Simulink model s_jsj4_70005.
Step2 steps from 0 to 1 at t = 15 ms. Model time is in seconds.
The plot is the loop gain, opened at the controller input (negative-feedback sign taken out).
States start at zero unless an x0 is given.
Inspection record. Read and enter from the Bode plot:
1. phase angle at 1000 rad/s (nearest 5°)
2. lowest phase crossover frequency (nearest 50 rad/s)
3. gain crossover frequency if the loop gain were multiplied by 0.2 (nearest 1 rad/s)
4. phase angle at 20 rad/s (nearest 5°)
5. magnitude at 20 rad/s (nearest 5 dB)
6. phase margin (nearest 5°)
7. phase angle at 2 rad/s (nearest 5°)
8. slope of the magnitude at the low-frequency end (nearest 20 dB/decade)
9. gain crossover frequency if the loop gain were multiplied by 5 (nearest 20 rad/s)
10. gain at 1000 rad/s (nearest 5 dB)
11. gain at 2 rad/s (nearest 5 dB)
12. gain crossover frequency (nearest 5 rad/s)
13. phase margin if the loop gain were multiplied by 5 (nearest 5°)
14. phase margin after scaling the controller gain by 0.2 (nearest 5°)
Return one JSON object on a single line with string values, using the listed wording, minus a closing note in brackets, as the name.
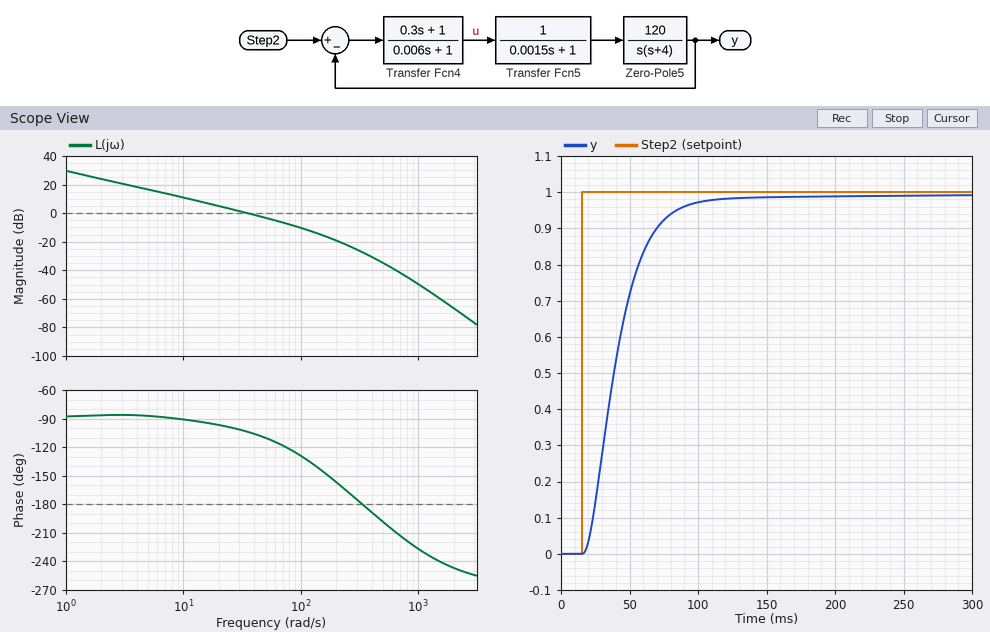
{"phase angle at 1000 rad/s": "-225°", "lowest phase crossover frequency": "350 rad/s", "gain crossover frequency if the loop gain were multiplied by 0.2": "7 rad/s", "phase angle at 20 rad/s": "-95°", "magnitude at 20 rad/s": "5 dB", "phase margin": "75°", "phase angle at 2 rad/s": "-85°", "slope of the magnitude at the low-frequency end": "-20 dB/decade", "gain crossover frequency if the loop gain were multiplied by 5": "140 rad/s", "gain at 1000 rad/s": "-50 dB", "gain at 2 rad/s": "25 dB", "gain crossover frequency": "35 rad/s", "phase margin if the loop gain were multiplied by 5": "40°", "phase margin after scaling the controller gain by 0.2": "90°"}
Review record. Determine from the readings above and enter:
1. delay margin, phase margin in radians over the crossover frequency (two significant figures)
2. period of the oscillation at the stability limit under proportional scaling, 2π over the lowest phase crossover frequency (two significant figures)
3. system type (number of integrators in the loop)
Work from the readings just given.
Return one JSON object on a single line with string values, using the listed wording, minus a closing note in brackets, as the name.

{"delay margin, phase margin in radians over the crossover frequency": "0.037 s", "period of the oscillation at the stability limit under proportional scaling, 2π over the lowest phase crossover frequency": "0.018 s", "system type": "1"}
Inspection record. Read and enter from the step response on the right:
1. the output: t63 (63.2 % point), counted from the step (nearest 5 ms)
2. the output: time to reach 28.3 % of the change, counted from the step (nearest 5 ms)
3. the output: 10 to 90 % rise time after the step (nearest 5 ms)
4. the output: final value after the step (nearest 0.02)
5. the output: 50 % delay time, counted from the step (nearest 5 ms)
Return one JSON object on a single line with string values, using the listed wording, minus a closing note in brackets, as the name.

{"the output: t63 (63.2 % point), counted from the step": "30 ms", "the output: time to reach 28.3 % of the change, counted from the step": "15 ms", "the output: 10 to 90 % rise time after the step": "45 ms", "the output: final value after the step": "1.00", "the output: 50 % delay time, counted from the step": "25 ms"}
